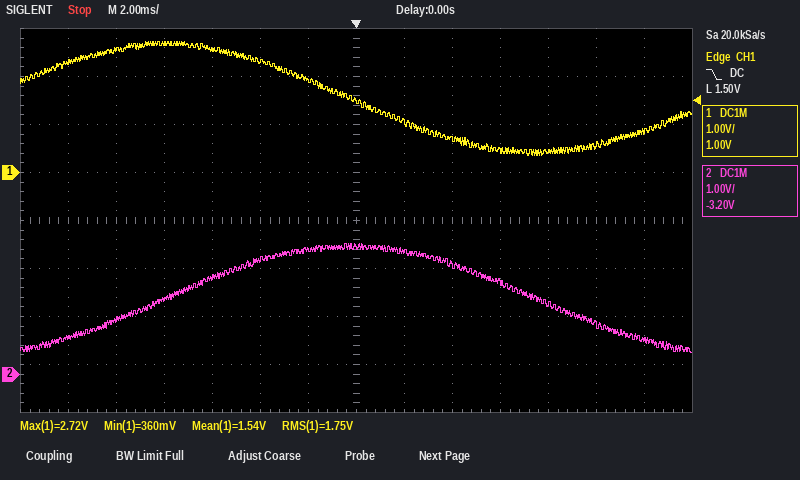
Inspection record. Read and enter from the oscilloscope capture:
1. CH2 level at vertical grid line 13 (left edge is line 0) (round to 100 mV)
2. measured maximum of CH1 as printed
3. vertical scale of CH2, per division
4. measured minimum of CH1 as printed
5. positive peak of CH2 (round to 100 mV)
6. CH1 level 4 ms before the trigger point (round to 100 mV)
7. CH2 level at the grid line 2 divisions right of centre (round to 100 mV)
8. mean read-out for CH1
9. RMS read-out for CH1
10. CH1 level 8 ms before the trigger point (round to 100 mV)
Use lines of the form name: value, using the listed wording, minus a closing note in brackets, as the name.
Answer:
CH2 level at vertical grid line 13 (left edge is line 0): 700 mV
measured maximum of CH1 as printed: 2.72 V
vertical scale of CH2, per division: 1 V
measured minimum of CH1 as printed: 360 mV
positive peak of CH2: 2.7 V
CH1 level 4 ms before the trigger point: 2.3 V
CH2 level at the grid line 2 divisions right of centre: 2.3 V
mean read-out for CH1: 1.54 V
RMS read-out for CH1: 1.75 V
CH1 level 8 ms before the trigger point: 2.7 V
